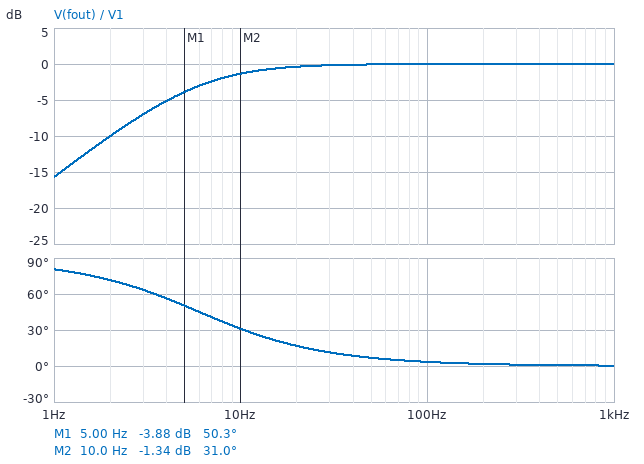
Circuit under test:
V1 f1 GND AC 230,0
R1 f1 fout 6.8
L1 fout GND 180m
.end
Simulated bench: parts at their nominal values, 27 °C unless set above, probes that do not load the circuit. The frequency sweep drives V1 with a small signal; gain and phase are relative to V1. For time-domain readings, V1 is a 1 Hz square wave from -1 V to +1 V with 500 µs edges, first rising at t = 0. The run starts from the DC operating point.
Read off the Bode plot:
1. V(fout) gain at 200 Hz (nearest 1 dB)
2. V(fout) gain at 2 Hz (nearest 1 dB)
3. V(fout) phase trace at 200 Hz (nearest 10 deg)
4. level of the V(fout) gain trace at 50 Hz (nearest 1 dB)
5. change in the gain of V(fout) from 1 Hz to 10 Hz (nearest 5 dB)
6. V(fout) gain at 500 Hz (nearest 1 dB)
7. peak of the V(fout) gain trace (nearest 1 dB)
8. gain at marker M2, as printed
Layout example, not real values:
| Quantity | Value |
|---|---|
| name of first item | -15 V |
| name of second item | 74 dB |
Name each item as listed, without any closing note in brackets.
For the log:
| Quantity | Value |
|---|---|
| V(fout) gain at 200 Hz | 0 dB |
| V(fout) gain at 2 Hz | -10 dB |
| V(fout) phase trace at 200 Hz | 0 deg |
| level of the V(fout) gain trace at 50 Hz | 0 dB |
| change in the gain of V(fout) from 1 Hz to 10 Hz | 15 dB |
| V(fout) gain at 500 Hz | 0 dB |
| peak of the V(fout) gain trace | 0 dB |
| gain at marker M2, as printed | -1.34 dB |
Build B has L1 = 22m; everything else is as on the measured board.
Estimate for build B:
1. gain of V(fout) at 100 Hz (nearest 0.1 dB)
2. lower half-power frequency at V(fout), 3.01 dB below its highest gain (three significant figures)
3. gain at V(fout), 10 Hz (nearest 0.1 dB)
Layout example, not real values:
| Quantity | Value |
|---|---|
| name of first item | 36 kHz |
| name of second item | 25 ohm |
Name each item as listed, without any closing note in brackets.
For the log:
| Quantity | Value |
|---|---|
| gain of V(fout) at 100 Hz | -0.9 dB |
| lower half-power frequency at V(fout), 3.01 dB below its highest gain | 49.2 Hz |
| gain at V(fout), 10 Hz | -14.0 dB |
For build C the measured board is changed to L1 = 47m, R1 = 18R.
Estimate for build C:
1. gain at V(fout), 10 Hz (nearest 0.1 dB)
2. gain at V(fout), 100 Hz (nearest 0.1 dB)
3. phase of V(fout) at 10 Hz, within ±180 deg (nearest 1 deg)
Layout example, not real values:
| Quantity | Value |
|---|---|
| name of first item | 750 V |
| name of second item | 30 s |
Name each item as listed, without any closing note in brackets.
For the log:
| Quantity | Value |
|---|---|
| gain at V(fout), 10 Hz | -15.8 dB |
| gain at V(fout), 100 Hz | -1.4 dB |
| phase of V(fout) at 10 Hz, within ±180 deg | 81 deg |
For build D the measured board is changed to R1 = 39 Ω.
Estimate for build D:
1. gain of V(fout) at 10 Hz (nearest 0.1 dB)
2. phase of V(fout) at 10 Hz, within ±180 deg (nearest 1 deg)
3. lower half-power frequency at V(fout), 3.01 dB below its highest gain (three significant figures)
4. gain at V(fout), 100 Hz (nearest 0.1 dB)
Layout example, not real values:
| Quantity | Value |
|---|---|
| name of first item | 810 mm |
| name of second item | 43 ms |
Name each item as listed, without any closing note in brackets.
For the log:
| Quantity | Value |
|---|---|
| gain of V(fout) at 10 Hz | -11.1 dB |
| phase of V(fout) at 10 Hz, within ±180 deg | 74 deg |
| lower half-power frequency at V(fout), 3.01 dB below its highest gain | 34.5 Hz |
| gain at V(fout), 100 Hz | -0.5 dB |
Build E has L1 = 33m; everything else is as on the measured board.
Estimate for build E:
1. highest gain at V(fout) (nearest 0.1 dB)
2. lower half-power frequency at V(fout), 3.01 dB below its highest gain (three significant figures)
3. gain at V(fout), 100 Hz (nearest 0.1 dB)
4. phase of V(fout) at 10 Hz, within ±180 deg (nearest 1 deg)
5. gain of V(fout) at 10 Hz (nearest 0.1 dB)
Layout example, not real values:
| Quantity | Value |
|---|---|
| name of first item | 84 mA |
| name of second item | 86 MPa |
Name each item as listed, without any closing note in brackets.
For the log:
| Quantity | Value |
|---|---|
| highest gain at V(fout) | 0 dB |
| lower half-power frequency at V(fout), 3.01 dB below its highest gain | 32.8 Hz |
| gain at V(fout), 100 Hz | -0.4 dB |
| phase of V(fout) at 10 Hz, within ±180 deg | 73 deg |
| gain of V(fout) at 10 Hz | -10.7 dB |
